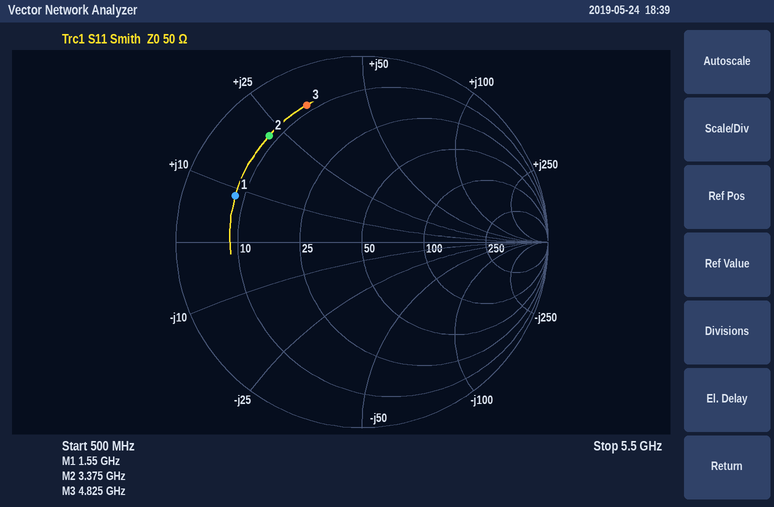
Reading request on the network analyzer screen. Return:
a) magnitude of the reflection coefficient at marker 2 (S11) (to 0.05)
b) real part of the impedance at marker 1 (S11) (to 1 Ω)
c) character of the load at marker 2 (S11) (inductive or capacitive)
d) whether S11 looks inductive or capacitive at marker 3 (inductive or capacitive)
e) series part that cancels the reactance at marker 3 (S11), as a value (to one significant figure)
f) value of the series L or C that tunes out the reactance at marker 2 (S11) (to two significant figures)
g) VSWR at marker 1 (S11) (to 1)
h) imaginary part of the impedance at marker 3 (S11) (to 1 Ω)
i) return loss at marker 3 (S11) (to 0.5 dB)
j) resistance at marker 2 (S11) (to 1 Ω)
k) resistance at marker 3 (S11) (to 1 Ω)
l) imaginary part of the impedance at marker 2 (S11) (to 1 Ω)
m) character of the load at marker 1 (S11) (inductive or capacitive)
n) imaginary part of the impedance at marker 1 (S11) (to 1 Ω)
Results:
0.75
8 Ω
inductive
inductive
1.0 pF
2.1 pF
6
+33 Ω
2.0 dB
8 Ω
8 Ω
+22 Ω
inductive
+9 Ω
